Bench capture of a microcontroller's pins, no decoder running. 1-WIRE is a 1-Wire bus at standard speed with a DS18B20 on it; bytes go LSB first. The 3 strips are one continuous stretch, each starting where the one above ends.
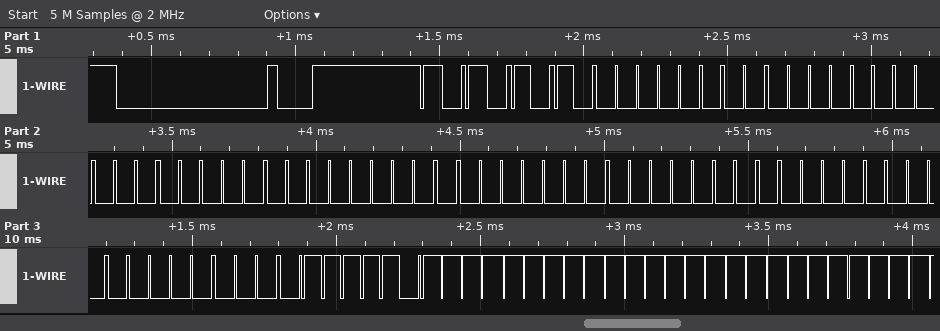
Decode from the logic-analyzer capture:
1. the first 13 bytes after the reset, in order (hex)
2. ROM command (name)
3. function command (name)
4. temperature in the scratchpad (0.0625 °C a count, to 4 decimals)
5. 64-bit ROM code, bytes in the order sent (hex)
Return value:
55 00 00 00 00 00 00 00 00 BE FF FF FF
Match ROM
Read Scratchpad
-0.0625 °C
00 00 00 00 00 00 00 00
